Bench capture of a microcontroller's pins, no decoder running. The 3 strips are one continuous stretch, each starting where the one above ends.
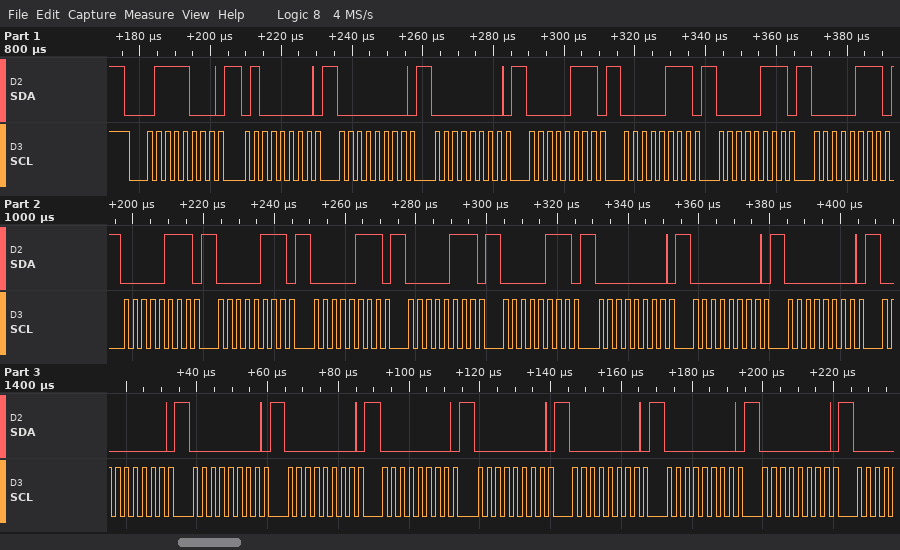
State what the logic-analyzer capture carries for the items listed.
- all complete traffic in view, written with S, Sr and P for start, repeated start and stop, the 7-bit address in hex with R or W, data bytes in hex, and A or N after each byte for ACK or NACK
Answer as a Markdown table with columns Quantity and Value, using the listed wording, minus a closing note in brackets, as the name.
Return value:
| Quantity | Value |
|---|---|
| all complete traffic in view, written with S, Sr and P for start, repeated start and stop, the 7-bit address in hex with R or W, data bytes in hex, and A or N after each byte for ACK or NACK | S 3CW A 40 A 00 A 00 A 07 A 07 A 07 A 07 A 07 A 07 A 07 A 07 A 07 A 00 A 00 A 00 A 00 A 00 A 00 A 00 A 00 A 00 A 00 A 00 A |
